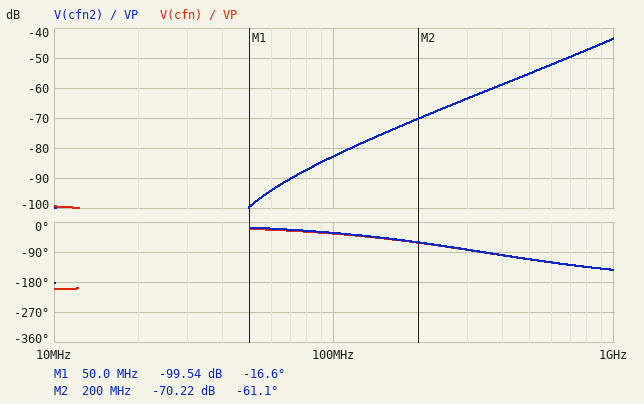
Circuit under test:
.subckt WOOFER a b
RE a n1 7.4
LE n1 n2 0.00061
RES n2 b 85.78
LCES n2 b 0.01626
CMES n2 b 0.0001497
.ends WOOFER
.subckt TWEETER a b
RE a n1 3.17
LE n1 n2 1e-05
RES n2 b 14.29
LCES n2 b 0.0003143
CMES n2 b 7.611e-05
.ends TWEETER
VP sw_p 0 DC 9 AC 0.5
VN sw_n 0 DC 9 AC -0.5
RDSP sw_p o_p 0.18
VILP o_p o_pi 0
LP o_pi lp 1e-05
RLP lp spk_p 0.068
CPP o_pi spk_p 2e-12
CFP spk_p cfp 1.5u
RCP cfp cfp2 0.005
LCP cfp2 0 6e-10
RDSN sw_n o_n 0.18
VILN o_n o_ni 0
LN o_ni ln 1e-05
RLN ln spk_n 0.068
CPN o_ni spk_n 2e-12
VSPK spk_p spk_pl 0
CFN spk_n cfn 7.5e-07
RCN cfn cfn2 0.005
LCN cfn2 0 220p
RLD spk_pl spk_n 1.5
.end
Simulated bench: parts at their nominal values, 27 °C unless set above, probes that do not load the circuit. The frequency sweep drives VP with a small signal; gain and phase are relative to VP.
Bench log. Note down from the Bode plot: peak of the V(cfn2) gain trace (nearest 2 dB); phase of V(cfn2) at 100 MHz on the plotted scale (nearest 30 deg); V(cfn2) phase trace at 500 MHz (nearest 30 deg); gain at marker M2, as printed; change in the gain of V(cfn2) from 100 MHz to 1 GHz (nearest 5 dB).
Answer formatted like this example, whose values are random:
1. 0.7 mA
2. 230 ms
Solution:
1. -44 dB
2. -30 deg
3. -120 deg
4. -70.22 dB
5. 40 dB
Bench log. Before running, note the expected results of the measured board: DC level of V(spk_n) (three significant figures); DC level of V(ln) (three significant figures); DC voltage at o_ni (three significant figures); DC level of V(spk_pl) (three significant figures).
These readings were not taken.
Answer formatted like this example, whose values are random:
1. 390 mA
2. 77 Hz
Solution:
1. 9.00 V
2. 9.00 V
3. 9.00 V
4. 9.00 V
